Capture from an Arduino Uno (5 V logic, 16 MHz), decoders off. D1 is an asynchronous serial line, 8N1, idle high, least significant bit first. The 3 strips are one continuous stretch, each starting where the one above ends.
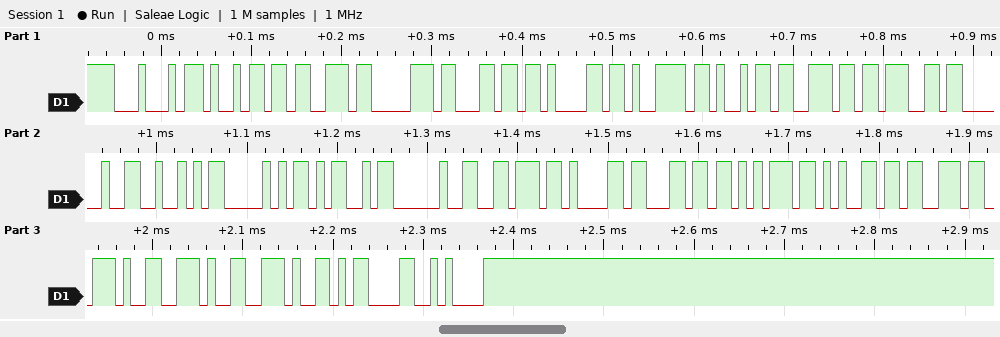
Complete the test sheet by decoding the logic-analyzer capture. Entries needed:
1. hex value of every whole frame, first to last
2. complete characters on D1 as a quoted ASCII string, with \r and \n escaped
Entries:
0x44 0x69 0x73 0x70 0x6C 0x61 0x79 0x69 0x6E 0x67 0x20 0x52 0x50 0x4D 0x20 0x76 0x61 0x6C 0x75 0x65 0x73 0x2E 0x2E 0x2E 0x0D 0x0A
"Displaying RPM values...\r\n"
